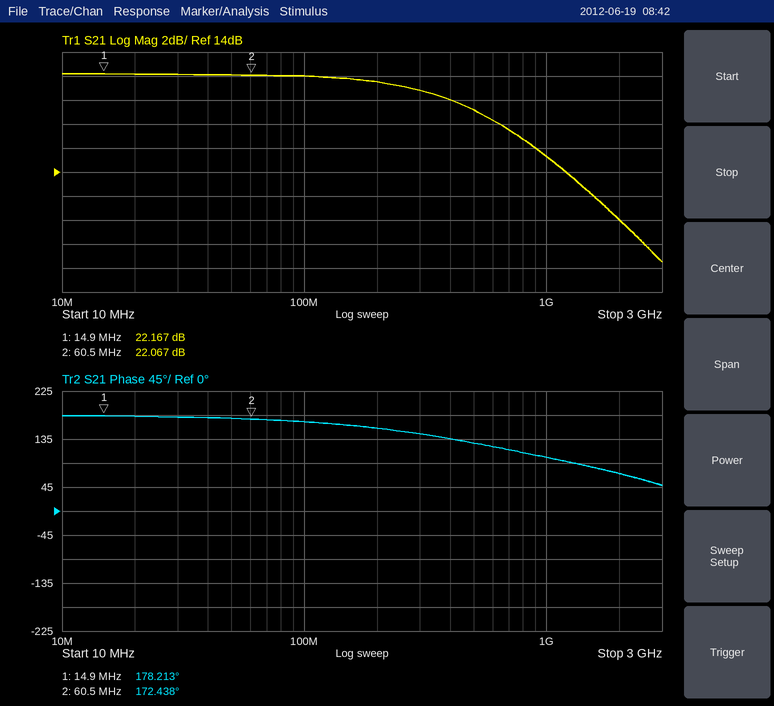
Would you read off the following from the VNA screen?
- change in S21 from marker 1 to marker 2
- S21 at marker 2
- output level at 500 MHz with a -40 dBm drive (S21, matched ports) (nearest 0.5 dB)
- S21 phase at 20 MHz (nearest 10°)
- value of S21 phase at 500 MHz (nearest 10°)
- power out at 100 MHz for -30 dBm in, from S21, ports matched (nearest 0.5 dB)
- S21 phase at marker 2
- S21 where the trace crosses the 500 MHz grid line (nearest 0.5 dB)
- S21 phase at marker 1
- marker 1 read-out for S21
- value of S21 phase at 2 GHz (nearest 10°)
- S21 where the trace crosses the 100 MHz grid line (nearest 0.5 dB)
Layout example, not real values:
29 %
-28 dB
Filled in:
-0.100 dB
22.067 dB
-21.0 dBm
180°
130°
-8.0 dBm
172.438°
19.0 dB
178.213°
22.167 dB
70°
22.0 dB
